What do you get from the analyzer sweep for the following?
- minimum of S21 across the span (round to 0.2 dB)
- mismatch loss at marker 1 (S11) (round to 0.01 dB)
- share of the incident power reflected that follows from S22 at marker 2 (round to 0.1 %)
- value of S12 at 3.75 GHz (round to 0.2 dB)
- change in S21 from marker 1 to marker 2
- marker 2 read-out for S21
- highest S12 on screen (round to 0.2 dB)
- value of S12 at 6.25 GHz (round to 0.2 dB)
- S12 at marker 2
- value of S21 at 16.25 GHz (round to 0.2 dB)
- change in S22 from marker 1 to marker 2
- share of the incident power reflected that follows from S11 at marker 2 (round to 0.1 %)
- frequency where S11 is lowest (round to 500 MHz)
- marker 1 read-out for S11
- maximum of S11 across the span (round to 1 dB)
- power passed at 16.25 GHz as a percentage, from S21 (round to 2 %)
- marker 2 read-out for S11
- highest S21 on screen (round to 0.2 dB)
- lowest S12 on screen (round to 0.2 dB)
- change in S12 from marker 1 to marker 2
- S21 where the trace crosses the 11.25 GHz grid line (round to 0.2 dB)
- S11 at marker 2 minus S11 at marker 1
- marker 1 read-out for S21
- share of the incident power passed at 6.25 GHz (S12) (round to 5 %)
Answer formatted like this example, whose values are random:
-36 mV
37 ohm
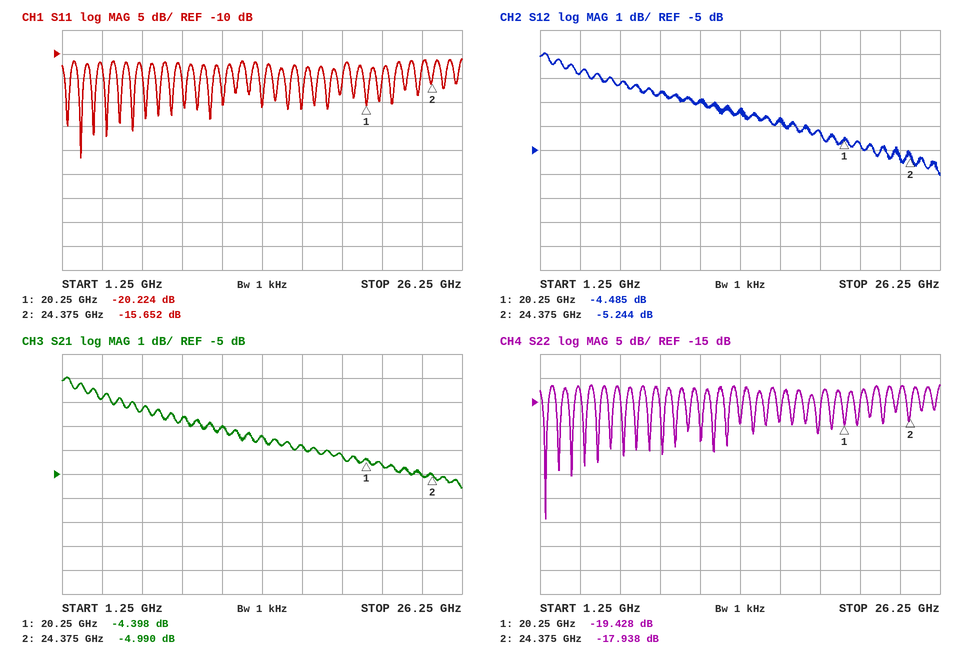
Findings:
-5.6 dB
0.04 dB
1.6 %
-1.8 dB
-0.592 dB
-4.990 dB
-1.0 dB
-2.2 dB
-5.244 dB
-3.8 dB
1.490 dB
2.7 %
2.5 GHz
-20.224 dB
-11 dB
42 %
-15.652 dB
-1.0 dB
-6.0 dB
-0.759 dB
-3.0 dB
4.572 dB
-4.398 dB
60 %
